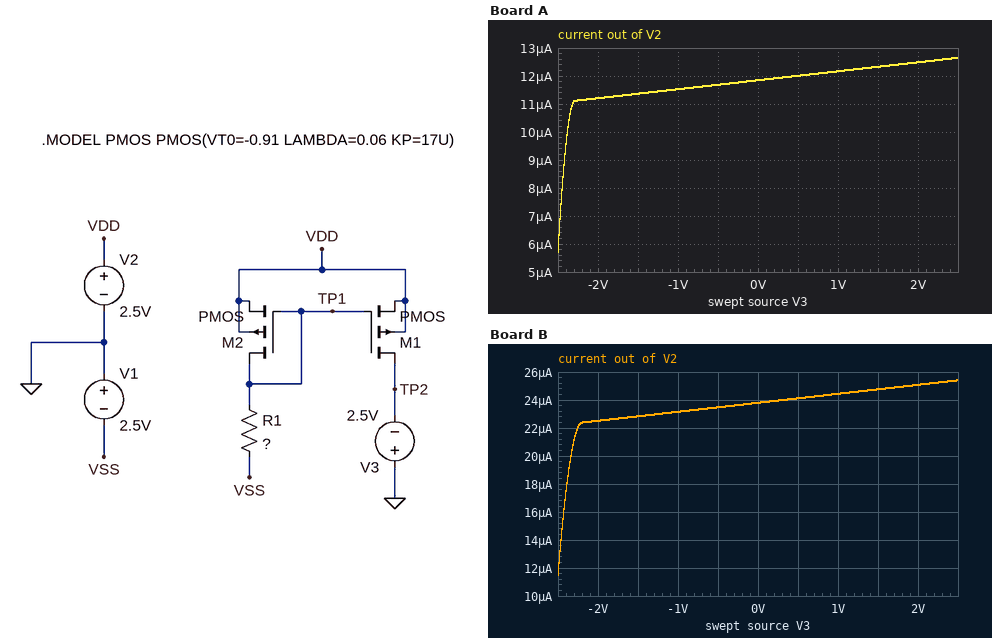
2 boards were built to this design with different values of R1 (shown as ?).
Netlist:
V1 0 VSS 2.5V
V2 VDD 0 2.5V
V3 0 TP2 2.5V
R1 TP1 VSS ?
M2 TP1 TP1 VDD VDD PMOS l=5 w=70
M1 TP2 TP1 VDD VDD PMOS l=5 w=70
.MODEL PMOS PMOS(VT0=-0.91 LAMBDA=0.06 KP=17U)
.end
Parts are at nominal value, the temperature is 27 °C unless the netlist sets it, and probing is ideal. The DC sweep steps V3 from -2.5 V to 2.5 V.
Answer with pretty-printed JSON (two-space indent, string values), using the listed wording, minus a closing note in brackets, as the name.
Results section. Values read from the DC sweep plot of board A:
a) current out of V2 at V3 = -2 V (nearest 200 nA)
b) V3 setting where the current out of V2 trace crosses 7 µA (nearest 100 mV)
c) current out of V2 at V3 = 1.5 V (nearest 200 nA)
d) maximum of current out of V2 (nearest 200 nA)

{
  "current out of V2 at V3 = -2 V": "11.2 µA",
  "V3 setting where the current out of V2 trace crosses 7 µA": "-2.5 V",
  "current out of V2 at V3 = 1.5 V": "12.4 µA",
  "maximum of current out of V2": "12.6 µA"
}
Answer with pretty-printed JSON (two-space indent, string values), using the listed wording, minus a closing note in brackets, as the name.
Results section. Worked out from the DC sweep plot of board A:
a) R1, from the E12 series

{
  "R1, from the E12 series": "680 kΩ"
}
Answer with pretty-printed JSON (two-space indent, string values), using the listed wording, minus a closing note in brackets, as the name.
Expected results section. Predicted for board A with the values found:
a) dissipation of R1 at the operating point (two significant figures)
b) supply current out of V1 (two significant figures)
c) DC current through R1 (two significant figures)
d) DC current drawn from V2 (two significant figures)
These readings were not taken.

{
  "dissipation of R1 at the operating point": "22 µW",
  "supply current out of V1": "5.7 µA",
  "DC current through R1": "5.7 µA",
  "DC current drawn from V2": "13 µA"
}
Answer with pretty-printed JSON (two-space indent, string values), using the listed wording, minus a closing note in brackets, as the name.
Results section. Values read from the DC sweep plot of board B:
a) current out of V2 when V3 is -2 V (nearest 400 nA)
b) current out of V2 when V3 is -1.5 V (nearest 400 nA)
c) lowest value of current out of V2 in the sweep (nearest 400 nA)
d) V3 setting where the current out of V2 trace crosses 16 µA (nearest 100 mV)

{
  "current out of V2 when V3 is -2 V": "22.4 µA",
  "current out of V2 when V3 is -1.5 V": "22.8 µA",
  "lowest value of current out of V2 in the sweep": "11.6 µA",
  "V3 setting where the current out of V2 trace crosses 16 µA": "-2.4 V"
}
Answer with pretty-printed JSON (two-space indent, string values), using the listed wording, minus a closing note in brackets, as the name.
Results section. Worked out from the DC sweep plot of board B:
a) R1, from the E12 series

{
  "R1, from the E12 series": "330 kΩ"
}
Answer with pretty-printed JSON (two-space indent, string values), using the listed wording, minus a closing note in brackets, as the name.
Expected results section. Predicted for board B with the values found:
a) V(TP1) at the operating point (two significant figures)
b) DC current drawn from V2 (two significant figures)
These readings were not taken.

{
  "V(TP1) at the operating point": "1.3 V",
  "DC current drawn from V2": "25 µA"
}
